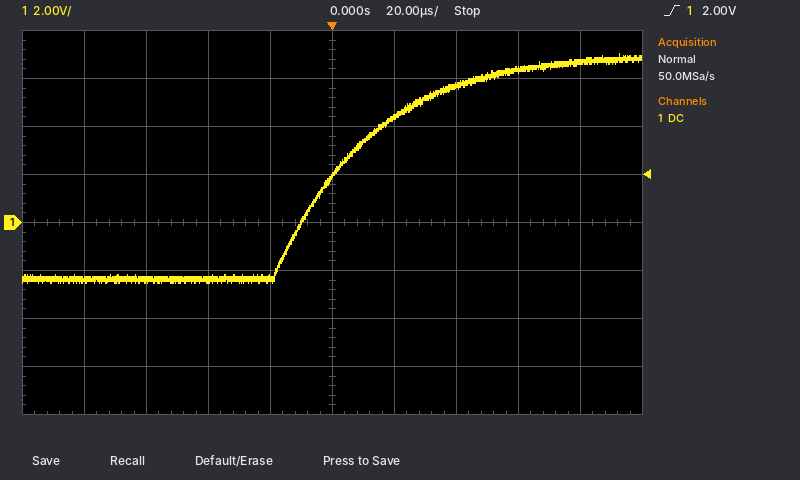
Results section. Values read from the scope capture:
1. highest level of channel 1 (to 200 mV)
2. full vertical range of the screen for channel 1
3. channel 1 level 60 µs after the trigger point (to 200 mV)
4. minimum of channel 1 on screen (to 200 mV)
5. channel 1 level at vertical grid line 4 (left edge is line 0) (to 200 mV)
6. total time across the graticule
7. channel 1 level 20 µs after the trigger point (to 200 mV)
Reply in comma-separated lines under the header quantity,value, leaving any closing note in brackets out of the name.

quantity,value
highest level of channel 1,7.0 V
full vertical range of the screen for channel 1,16 V
channel 1 level 60 µs after the trigger point,6.4 V
minimum of channel 1 on screen,-2.4 V
channel 1 level at vertical grid line 4 (left edge is line 0),-2.4 V
total time across the graticule,200 µs
channel 1 level 20 µs after the trigger point,4.4 V
